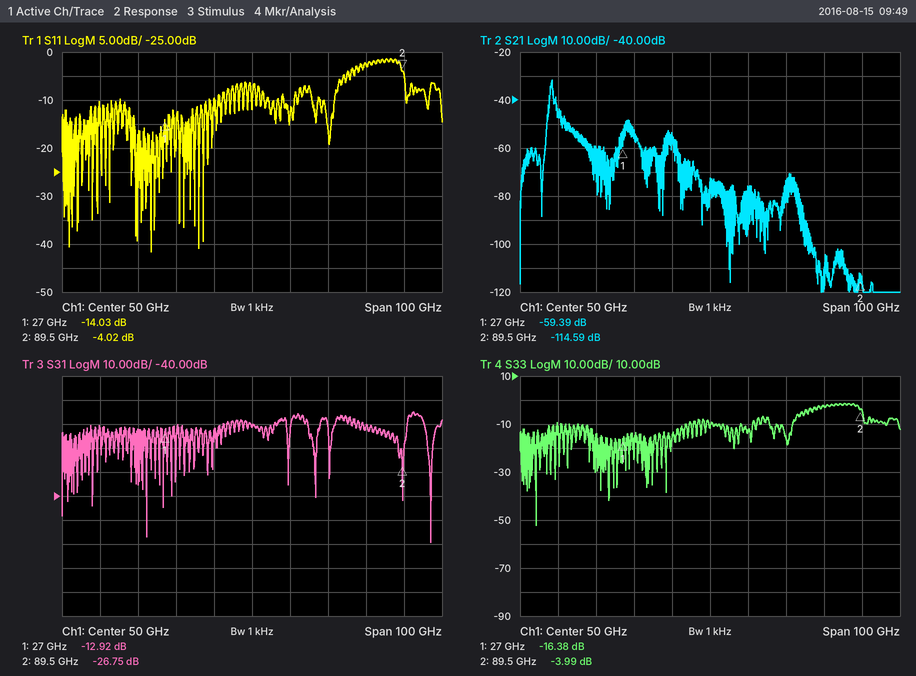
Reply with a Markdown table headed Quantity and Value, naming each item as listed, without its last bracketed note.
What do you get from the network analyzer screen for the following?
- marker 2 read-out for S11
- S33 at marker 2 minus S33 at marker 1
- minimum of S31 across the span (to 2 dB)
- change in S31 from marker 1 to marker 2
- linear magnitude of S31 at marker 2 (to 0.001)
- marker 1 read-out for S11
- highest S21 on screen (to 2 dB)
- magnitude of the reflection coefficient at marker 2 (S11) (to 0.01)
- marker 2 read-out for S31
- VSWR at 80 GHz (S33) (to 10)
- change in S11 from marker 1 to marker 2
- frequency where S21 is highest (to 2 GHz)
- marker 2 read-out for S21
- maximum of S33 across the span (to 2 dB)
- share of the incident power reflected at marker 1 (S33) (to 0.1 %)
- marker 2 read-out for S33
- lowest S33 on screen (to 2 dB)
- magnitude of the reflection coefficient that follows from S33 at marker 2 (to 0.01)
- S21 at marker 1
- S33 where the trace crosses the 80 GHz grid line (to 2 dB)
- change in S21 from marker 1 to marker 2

| Quantity | Value |
|---|---|
| marker 2 read-out for S11 | -4.02 dB |
| S33 at marker 2 minus S33 at marker 1 | 12.39 dB |
| minimum of S31 across the span | -60 dB |
| change in S31 from marker 1 to marker 2 | -13.83 dB |
| linear magnitude of S31 at marker 2 | 0.046 |
| marker 1 read-out for S11 | -14.03 dB |
| highest S21 on screen | -32 dB |
| magnitude of the reflection coefficient at marker 2 (S11) | 0.63 |
| marker 2 read-out for S31 | -26.75 dB |
| VSWR at 80 GHz (S33) | 10 |
| change in S11 from marker 1 to marker 2 | 10.01 dB |
| frequency where S21 is highest | 8 GHz |
| marker 2 read-out for S21 | -114.59 dB |
| maximum of S33 across the span | -2 dB |
| share of the incident power reflected at marker 1 (S33) | 2.3 % |
| marker 2 read-out for S33 | -3.99 dB |
| lowest S33 on screen | -52 dB |
| magnitude of the reflection coefficient that follows from S33 at marker 2 | 0.63 |
| S21 at marker 1 | -59.39 dB |
| S33 where the trace crosses the 80 GHz grid line | -2 dB |
| change in S21 from marker 1 to marker 2 | -55.20 dB |
